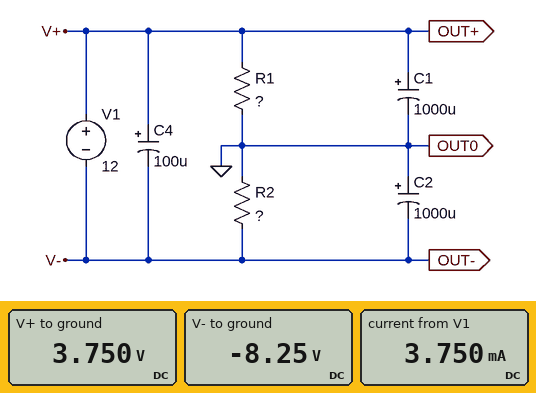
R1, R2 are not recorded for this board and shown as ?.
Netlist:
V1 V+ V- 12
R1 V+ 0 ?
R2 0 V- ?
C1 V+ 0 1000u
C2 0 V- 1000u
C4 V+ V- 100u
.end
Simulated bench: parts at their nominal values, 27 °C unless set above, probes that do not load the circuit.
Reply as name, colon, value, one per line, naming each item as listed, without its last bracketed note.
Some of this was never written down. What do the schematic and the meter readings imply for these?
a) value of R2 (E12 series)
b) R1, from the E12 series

value of R2: 2.2 kΩ
R1, from the E12 series: 1 kΩ
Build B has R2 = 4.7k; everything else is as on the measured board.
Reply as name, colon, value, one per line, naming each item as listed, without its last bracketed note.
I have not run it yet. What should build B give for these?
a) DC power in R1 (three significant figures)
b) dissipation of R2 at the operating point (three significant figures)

DC power in R1: 4.43 mW
dissipation of R2 at the operating point: 20.8 mW
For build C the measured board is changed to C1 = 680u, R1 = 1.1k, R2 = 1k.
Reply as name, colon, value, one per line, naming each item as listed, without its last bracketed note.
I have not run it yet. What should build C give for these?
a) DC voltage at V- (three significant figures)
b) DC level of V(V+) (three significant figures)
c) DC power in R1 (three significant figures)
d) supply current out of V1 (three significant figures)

DC voltage at V-: -5.71 V
DC level of V(V+): 6.29 V
DC power in R1: 35.9 mW
supply current out of V1: 5.71 mA
